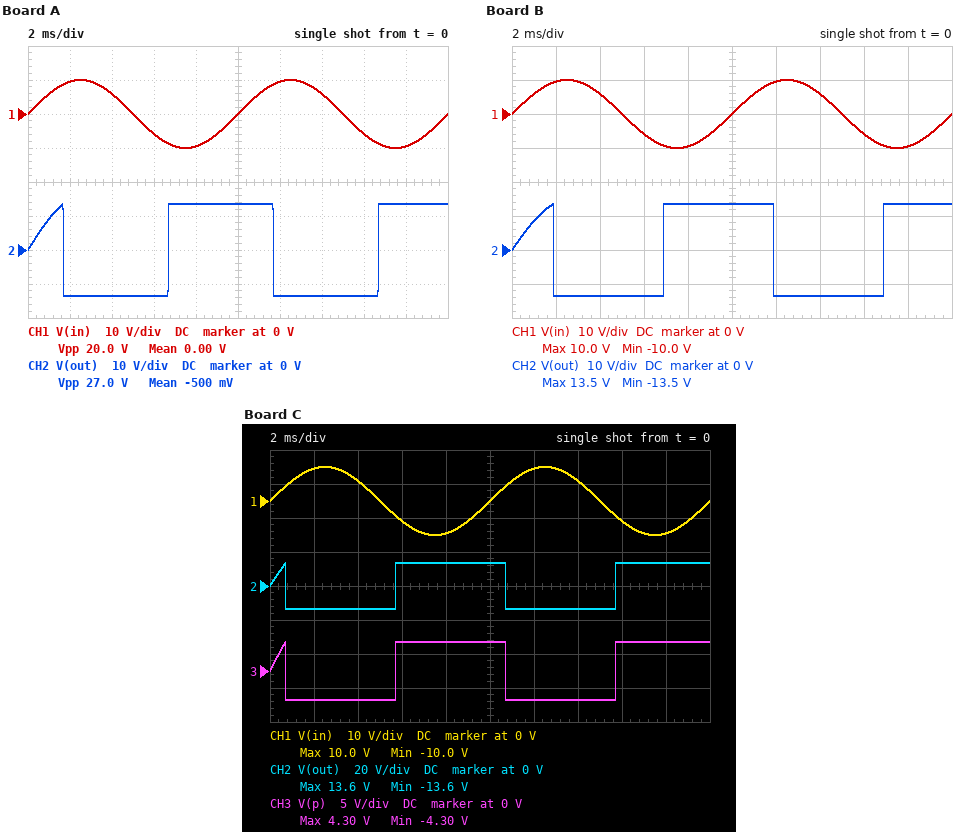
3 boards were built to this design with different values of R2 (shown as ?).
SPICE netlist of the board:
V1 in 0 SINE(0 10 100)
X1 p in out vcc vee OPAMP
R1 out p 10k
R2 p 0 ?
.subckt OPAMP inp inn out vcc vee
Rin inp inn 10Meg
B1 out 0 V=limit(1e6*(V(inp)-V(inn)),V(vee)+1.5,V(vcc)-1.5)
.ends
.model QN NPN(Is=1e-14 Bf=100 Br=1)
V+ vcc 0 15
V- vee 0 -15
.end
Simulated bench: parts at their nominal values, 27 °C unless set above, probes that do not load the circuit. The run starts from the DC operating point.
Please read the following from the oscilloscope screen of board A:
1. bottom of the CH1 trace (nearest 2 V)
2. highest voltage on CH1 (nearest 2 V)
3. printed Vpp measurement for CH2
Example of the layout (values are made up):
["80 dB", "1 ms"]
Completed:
["-10 V", "10 V", "27.0 V"]
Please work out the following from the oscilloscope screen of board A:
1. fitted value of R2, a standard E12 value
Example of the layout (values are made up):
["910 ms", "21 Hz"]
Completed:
["18 kΩ"]
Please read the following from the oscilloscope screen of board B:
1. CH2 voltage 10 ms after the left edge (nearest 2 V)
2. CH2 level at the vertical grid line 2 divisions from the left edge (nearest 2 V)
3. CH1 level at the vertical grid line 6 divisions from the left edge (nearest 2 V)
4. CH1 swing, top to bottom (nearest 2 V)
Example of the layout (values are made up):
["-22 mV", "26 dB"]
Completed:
["14 V", "-14 V", "10 V", "20 V"]
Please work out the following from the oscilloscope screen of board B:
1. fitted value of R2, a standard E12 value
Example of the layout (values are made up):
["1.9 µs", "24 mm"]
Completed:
["22 kΩ"]
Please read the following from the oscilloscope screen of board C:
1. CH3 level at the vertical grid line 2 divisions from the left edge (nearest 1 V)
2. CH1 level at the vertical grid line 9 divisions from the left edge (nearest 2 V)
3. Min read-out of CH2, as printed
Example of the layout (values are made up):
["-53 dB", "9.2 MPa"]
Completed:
["-4 V", "-10 V", "-13.6 V"]
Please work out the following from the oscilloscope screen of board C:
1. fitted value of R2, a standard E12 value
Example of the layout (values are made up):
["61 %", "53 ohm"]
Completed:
["4.7 kΩ"]
